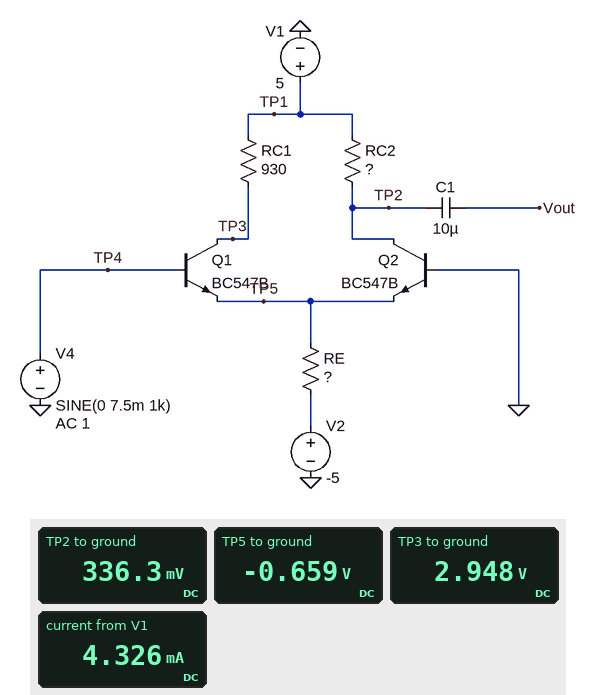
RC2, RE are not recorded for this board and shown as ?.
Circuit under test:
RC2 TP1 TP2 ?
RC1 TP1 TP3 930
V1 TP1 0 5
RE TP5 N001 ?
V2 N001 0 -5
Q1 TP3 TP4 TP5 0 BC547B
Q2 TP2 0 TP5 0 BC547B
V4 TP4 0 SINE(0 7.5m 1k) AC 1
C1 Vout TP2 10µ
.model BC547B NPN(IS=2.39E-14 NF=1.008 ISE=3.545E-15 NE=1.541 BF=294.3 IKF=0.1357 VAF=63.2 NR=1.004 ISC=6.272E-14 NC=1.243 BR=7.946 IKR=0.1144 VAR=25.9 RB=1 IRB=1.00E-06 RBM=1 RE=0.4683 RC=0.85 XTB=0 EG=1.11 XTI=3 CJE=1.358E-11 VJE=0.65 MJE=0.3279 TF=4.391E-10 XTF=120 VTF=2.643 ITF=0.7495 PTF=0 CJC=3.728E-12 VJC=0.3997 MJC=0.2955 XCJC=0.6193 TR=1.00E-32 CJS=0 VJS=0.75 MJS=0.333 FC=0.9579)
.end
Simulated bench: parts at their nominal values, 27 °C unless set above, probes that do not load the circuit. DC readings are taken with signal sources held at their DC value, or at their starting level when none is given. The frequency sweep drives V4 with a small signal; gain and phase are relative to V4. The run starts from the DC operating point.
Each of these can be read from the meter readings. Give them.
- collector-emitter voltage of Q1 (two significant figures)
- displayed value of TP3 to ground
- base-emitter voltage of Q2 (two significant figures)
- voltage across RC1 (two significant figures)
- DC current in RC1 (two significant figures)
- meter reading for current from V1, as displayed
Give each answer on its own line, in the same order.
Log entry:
3.6 V
2.948 V
660 mV
2.1 V
2.2 mA
4.326 mA
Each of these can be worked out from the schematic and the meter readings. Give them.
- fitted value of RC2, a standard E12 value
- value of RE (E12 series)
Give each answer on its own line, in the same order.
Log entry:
2.2 kΩ
1 kΩ
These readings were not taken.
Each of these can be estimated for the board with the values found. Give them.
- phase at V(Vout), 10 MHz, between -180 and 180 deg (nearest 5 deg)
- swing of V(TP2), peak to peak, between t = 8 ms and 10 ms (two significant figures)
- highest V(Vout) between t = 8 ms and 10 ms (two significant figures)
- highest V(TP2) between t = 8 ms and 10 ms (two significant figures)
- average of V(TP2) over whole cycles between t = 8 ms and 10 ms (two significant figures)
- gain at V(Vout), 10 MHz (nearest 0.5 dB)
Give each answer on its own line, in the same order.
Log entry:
-25 deg
1.2 V
610 mV
940 mV
340 mV
37.5 dB
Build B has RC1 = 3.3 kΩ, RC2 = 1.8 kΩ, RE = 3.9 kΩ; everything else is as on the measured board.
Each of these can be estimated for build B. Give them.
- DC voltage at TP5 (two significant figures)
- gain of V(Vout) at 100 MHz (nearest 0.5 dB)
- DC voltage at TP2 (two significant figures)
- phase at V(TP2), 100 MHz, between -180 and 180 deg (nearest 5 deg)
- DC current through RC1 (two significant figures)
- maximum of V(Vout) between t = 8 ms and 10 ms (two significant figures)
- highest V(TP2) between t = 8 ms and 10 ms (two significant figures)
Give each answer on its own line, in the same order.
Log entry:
-620 mV
18.0 dB
4.0 V
-65 deg
560 µA
140 mV
4.1 V
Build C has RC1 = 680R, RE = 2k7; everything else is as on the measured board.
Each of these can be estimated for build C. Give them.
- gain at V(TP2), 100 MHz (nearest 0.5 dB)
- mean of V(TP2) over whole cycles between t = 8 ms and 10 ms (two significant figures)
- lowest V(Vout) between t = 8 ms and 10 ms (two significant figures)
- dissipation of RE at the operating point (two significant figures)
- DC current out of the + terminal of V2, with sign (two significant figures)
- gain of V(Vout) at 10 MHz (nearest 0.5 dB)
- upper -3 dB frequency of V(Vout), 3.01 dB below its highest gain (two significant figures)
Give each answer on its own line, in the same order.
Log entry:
21.0 dB
3.2 V
-240 mV
7.1 mW
-1.6 mA
30.0 dB
37 MHz
